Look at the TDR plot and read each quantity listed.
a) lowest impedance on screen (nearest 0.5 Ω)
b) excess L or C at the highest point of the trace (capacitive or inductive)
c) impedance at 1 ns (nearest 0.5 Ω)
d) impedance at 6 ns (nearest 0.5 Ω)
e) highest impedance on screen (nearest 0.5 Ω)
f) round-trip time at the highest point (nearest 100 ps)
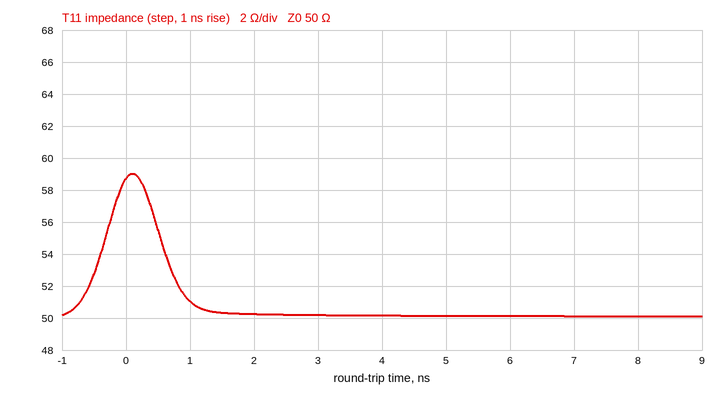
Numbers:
50.0 Ω
inductive
51.0 Ω
50.0 Ω
59.0 Ω
100 ps
